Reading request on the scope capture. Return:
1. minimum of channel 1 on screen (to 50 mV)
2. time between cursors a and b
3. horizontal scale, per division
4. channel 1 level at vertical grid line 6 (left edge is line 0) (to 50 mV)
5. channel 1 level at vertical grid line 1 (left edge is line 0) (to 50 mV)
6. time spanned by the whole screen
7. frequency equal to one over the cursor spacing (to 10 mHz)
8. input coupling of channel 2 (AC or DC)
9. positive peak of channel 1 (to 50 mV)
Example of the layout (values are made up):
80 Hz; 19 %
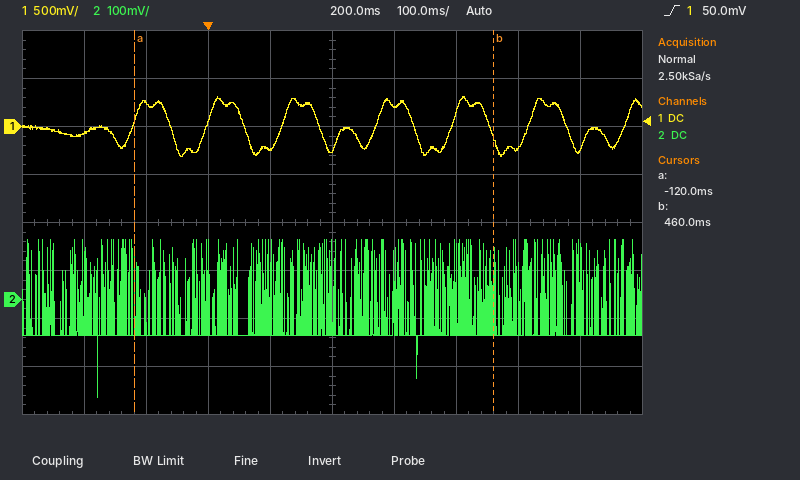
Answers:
-300 mV; 580 ms; 100 ms; 200 mV; -50 mV; 1 s; 1.72 Hz; DC; 300 mV
